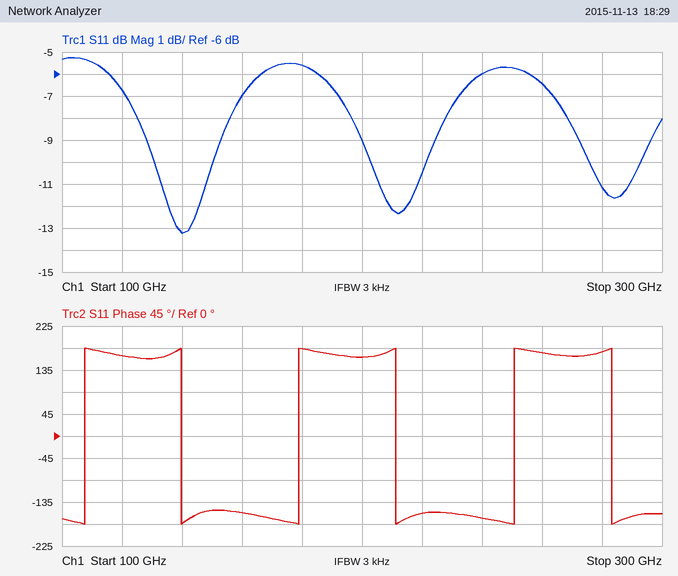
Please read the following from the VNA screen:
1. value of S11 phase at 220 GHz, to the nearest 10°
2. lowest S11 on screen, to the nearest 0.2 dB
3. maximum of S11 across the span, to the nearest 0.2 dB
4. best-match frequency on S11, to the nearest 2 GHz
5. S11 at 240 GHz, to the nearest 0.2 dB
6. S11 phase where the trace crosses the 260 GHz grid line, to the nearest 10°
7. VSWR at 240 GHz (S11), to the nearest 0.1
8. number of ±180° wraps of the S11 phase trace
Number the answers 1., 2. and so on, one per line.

1. -160°
2. -13.2 dB
3. -5.2 dB
4. 140 GHz
5. -6.0 dB
6. 170°
7. 3.0
8. 6
